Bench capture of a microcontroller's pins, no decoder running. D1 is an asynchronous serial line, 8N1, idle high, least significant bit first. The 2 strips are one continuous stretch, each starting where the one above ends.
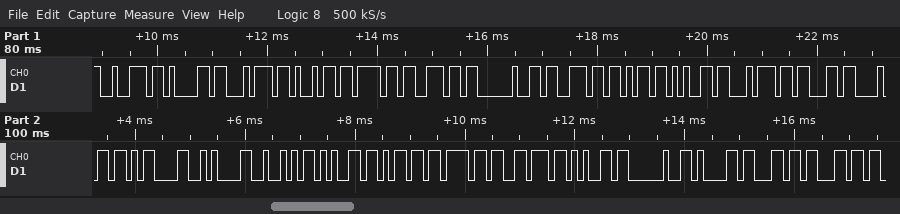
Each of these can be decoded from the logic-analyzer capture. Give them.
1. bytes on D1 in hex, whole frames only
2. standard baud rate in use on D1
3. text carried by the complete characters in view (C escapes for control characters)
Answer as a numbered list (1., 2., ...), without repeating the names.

1. 72 61 74 69 6F 6E 20 73 6B 65 74 63 68 0D 0A 52 65 6D 6F 76 65 20 61 6C 6C
2. 9600 baud
3. "ration sketch\r\nRemove all"
